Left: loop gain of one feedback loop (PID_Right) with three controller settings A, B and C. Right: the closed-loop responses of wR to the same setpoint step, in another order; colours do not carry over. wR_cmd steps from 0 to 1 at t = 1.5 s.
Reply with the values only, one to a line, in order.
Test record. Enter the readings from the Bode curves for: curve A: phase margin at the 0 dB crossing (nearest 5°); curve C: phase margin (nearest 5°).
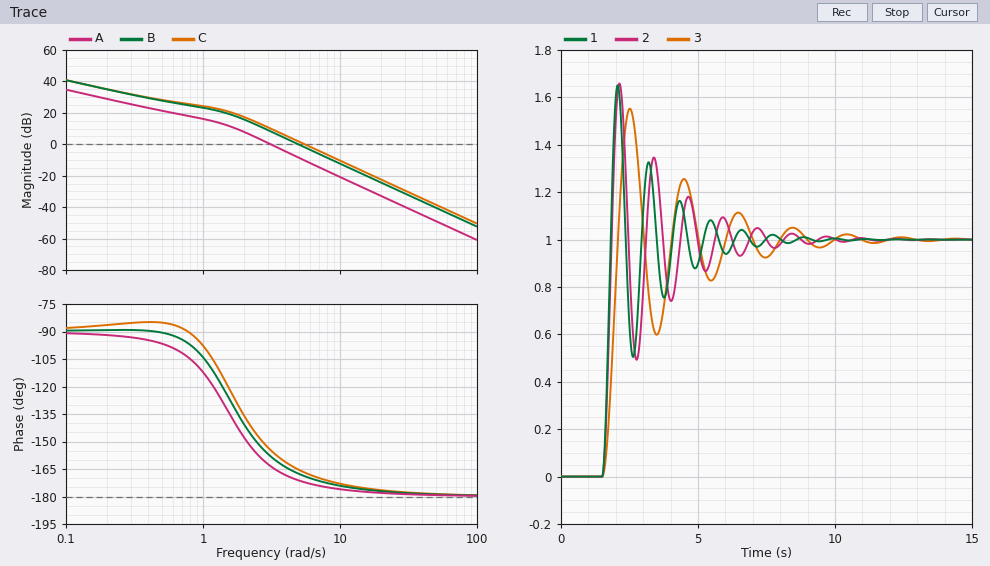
15°
15°
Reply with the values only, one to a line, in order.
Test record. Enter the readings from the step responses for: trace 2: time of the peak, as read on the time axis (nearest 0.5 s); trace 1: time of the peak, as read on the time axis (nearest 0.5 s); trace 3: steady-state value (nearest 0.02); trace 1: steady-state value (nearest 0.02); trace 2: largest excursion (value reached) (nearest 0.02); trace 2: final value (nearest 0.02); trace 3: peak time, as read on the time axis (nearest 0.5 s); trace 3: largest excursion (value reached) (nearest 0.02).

2.0 s
2.0 s
1.00
1.00
1.66
1.00
2.5 s
1.56
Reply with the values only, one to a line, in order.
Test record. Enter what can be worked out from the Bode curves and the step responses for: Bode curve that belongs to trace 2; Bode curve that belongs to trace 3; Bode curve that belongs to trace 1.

B
A
C
